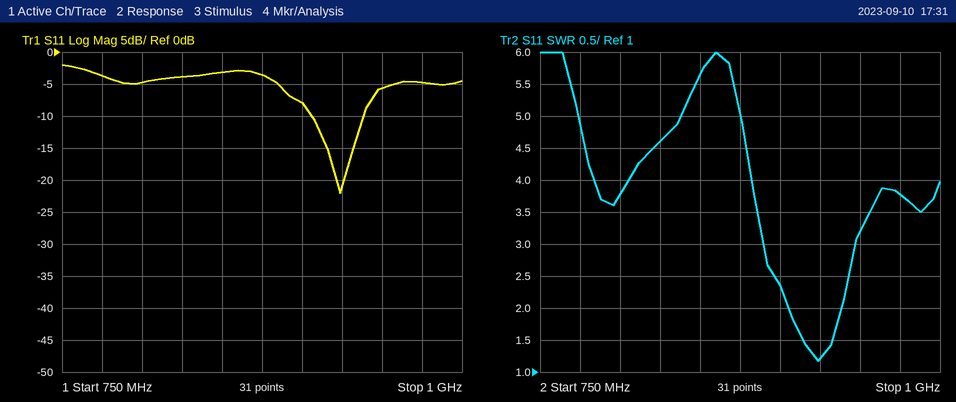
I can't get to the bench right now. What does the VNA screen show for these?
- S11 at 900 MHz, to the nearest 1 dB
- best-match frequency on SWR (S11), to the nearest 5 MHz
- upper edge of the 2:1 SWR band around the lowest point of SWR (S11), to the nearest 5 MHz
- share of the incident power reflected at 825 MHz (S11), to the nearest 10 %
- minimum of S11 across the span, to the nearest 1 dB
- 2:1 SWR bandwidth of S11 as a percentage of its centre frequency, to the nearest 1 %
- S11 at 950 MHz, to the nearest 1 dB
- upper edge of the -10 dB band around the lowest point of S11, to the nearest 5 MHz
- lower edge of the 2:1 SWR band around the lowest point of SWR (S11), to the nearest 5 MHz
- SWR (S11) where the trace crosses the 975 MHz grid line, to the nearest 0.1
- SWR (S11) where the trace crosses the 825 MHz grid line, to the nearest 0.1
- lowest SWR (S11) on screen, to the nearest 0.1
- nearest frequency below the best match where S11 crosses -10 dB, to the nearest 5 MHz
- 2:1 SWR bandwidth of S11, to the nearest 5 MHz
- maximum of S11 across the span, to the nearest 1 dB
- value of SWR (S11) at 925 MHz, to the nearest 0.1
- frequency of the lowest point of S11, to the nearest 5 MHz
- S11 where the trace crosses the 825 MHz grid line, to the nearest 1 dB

-8 dB
925 MHz
940 MHz
40 %
-22 dB
4 %
-6 dB
940 MHz
905 MHz
3.8
4.6
1.2
905 MHz
35 MHz
-2 dB
1.2
925 MHz
-4 dB
